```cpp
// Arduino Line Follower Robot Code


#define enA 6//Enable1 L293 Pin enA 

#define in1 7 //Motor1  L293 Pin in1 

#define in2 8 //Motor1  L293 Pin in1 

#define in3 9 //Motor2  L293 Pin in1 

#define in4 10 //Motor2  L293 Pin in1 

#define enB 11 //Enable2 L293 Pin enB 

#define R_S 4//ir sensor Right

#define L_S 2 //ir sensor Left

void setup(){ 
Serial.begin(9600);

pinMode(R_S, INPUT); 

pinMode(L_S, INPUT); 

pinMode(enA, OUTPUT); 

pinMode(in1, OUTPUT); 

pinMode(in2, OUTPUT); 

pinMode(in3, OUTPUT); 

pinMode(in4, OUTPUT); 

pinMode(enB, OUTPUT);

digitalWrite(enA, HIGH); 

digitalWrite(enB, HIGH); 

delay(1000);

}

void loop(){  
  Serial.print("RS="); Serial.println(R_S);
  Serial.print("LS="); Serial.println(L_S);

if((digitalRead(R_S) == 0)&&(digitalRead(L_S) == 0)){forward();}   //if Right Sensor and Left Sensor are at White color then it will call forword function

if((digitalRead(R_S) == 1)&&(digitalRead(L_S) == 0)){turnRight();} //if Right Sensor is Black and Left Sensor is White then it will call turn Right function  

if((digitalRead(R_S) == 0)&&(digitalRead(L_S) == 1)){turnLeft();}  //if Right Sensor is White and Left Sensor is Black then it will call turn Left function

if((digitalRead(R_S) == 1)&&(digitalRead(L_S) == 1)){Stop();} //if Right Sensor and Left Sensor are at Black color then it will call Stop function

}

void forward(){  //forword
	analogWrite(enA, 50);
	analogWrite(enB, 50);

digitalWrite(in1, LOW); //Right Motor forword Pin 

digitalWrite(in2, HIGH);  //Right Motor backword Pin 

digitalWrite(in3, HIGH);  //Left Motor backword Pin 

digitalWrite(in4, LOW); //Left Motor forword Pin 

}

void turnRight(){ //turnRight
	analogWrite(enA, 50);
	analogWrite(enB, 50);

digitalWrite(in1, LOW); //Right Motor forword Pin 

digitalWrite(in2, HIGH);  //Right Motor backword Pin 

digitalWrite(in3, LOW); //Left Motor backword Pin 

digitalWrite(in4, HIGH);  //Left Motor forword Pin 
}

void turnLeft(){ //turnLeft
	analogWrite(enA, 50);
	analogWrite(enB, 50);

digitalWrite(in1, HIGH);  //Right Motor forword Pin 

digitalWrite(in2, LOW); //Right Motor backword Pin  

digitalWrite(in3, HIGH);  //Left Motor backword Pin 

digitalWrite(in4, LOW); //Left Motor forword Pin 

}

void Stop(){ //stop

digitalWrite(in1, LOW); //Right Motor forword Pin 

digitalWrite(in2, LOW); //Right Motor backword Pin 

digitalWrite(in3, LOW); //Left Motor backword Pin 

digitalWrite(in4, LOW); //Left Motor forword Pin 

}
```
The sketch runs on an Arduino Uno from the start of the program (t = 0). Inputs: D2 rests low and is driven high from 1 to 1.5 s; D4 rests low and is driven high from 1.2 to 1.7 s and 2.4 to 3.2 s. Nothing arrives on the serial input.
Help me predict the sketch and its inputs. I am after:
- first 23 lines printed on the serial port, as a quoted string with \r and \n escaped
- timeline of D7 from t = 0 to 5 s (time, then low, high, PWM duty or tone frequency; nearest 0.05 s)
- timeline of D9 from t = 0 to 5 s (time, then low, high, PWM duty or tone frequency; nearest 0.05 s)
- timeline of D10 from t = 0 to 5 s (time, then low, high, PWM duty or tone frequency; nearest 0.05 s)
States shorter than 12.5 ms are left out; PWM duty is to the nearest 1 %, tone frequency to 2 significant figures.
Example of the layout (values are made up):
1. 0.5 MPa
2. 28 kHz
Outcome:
1. "RS=4\r\nLS=2\r\nRS=4\r\nLS=2\r\nRS=4\r\nLS=2\r\nRS=4\r\nLS=2\r\nRS=4\r\nLS=2\r\nRS=4\r\nLS=2\r\nRS=4\r\nLS=2\r\nRS=4\r\nLS=2\r\nRS=4\r\nLS=2\r\nRS=4\r\nLS=2\r\nRS=4\r\nLS=2\r\nRS=4\r\n"
2. 0 s low; 1 s high; 1.2 s low
3. 0 s low; 1 s high; 1.2 s low; 1.7 s high; 2.4 s low; 3.2 s high
4. 0 s low; 1.5 s high; 1.7 s low; 2.4 s high; 3.2 s low
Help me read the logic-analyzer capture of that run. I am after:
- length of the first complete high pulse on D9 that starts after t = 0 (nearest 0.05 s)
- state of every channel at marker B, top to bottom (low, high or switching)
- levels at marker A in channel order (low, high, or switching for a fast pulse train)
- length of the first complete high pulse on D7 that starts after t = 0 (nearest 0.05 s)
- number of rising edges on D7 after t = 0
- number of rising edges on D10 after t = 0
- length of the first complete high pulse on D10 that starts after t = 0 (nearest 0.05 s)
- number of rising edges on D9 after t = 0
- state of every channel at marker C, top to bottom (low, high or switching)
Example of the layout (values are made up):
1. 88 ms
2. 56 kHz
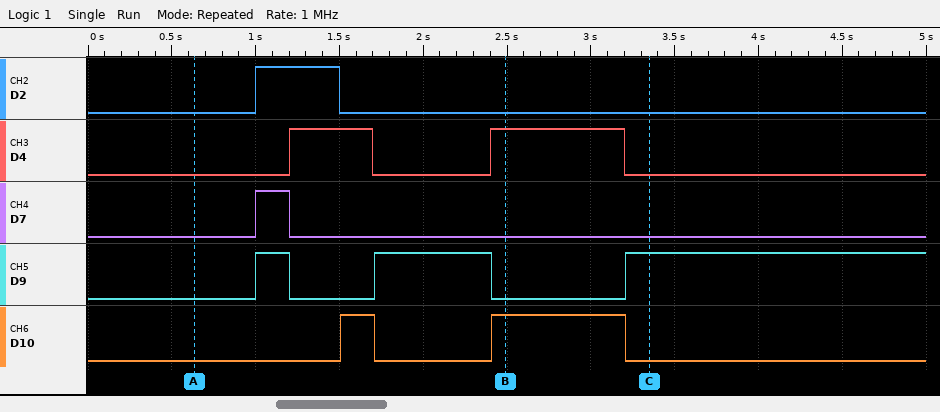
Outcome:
1. 0.20 s
2. D2 low, D4 high, D7 low, D9 low, D10 high
3. D2 low, D4 low, D7 low, D9 low, D10 low
4. 0.20 s
5. 1
6. 2
7. 0.20 s
8. 3
9. D2 low, D4 low, D7 low, D9 high, D10 low
